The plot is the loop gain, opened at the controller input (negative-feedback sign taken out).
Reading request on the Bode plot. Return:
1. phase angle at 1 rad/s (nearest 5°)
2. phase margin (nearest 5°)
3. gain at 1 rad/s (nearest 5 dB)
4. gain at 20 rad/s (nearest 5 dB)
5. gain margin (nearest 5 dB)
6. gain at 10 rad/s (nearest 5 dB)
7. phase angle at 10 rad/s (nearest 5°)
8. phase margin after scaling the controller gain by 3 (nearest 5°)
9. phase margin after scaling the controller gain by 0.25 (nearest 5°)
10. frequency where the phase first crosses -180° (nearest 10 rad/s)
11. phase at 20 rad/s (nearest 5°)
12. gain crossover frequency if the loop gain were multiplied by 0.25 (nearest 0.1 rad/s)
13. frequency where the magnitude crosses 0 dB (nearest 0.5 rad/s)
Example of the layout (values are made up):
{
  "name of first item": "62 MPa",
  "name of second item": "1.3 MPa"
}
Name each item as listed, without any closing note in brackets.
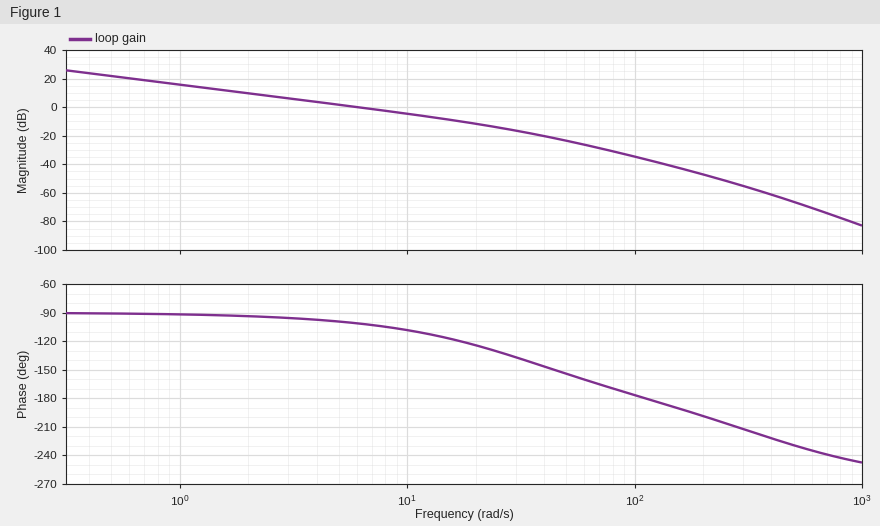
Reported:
{
  "phase angle at 1 rad/s": "-90°",
  "phase margin": "80°",
  "gain at 1 rad/s": "15 dB",
  "gain at 20 rad/s": "-10 dB",
  "gain margin": "35 dB",
  "gain at 10 rad/s": "-5 dB",
  "phase angle at 10 rad/s": "-110°",
  "phase margin after scaling the controller gain by 3": "60°",
  "phase margin after scaling the controller gain by 0.25": "85°",
  "frequency where the phase first crosses -180°": "110 rad/s",
  "phase at 20 rad/s": "-125°",
  "gain crossover frequency if the loop gain were multiplied by 0.25": "1.5 rad/s",
  "frequency where the magnitude crosses 0 dB": "6.0 rad/s"
}
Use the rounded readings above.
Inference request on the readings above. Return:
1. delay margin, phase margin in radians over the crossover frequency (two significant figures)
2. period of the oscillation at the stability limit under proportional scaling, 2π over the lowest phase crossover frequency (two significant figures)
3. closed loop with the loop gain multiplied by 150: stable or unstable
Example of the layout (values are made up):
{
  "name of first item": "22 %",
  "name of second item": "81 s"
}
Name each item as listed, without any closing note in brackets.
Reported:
{
  "delay margin, phase margin in radians over the crossover frequency": "0.23 s",
  "period of the oscillation at the stability limit under proportional scaling, 2π over the lowest phase crossover frequency": "0.057 s",
  "closed loop with the loop gain multiplied by 150: stable or unstable": "unstable"
}
